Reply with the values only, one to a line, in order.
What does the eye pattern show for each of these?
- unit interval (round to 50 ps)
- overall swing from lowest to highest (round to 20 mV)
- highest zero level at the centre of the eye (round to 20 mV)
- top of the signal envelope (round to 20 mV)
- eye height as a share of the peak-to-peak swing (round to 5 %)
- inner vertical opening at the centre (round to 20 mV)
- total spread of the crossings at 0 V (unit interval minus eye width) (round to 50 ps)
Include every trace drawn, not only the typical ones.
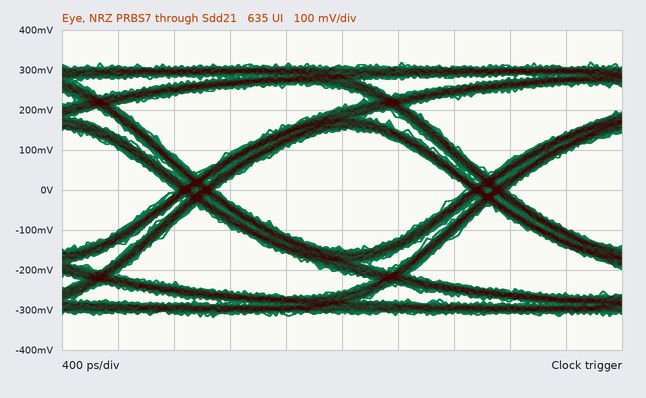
2.10 ns
640 mV
-140 mV
320 mV
45 %
300 mV
300 ps
